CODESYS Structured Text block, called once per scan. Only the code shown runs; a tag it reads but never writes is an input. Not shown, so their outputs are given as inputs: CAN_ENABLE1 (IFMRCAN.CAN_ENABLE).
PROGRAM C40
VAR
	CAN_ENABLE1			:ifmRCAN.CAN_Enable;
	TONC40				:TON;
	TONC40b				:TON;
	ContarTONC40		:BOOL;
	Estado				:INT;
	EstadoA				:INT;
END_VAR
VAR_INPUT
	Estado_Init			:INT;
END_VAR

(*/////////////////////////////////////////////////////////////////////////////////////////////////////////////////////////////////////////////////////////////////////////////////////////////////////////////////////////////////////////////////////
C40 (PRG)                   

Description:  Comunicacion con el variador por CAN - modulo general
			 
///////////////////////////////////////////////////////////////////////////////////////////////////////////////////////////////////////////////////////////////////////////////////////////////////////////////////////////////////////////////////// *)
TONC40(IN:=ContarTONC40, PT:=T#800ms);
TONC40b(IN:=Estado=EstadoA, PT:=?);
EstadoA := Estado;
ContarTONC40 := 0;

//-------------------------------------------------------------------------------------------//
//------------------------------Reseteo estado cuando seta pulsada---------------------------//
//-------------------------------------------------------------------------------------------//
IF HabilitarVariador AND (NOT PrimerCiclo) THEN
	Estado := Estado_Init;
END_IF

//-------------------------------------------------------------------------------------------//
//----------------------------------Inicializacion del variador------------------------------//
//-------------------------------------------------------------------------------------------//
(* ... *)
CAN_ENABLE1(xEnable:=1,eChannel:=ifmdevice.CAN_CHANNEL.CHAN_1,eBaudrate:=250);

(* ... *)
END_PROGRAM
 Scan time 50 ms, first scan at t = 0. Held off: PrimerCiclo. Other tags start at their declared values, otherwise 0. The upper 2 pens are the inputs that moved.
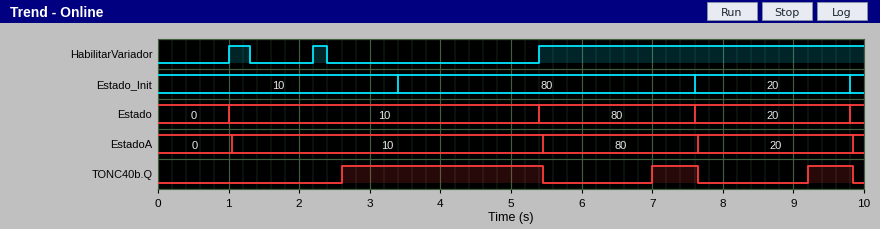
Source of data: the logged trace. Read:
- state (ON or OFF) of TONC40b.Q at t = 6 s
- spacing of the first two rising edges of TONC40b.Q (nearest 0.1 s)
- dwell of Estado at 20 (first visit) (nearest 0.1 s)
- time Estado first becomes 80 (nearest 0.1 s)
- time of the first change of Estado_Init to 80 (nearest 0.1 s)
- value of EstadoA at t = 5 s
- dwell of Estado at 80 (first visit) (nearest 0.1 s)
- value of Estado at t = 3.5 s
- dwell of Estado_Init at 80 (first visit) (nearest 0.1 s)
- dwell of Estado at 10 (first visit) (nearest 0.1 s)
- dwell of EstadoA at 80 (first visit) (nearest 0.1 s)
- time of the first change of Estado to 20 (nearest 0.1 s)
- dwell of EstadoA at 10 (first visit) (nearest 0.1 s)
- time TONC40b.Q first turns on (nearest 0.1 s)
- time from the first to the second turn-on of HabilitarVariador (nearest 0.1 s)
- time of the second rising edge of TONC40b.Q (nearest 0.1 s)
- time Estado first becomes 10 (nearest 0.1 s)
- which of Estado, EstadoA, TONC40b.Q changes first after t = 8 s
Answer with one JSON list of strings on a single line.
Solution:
["OFF", "4.4 s", "2.2 s", "5.4 s", "3.4 s", "10", "2.2 s", "10", "4.2 s", "4.4 s", "2.2 s", "7.6 s", "4.4 s", "2.6 s", "1.2 s", "7.0 s", "1.0 s", "TONC40b.Q"]
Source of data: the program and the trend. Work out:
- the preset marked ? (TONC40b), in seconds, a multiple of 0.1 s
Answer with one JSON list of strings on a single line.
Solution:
["1.5 s"]
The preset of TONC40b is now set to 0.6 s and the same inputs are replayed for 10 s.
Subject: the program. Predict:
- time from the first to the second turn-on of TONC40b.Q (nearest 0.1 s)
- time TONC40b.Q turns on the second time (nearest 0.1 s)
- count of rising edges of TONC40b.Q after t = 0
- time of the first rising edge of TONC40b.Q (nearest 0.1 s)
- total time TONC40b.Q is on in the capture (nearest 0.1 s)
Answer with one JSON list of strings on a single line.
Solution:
["1.1 s", "1.7 s", "4", "0.6 s", "7.3 s"]
